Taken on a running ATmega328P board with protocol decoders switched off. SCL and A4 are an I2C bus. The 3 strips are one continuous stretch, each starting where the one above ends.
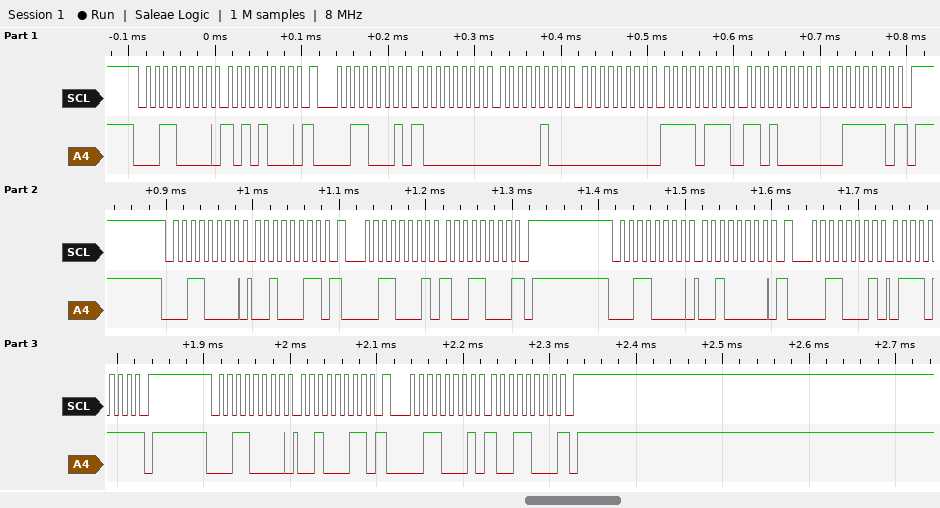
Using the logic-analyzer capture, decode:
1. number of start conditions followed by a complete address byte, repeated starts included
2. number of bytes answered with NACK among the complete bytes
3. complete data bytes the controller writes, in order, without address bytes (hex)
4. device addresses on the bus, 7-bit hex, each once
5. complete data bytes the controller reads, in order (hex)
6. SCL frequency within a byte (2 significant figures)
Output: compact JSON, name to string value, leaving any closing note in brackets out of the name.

{"number of start conditions followed by a complete address byte, repeated starts included": "8", "number of bytes answered with NACK among the complete bytes": "4", "complete data bytes the controller writes, in order, without address bytes": "A8 23 20 23", "device addresses on the bus, 7-bit hex, each once": "0x18", "complete data bytes the controller reads, in order": "80 04 00 F7 D0 3E 98 77 98", "SCL frequency within a byte": "100 kHz"}
